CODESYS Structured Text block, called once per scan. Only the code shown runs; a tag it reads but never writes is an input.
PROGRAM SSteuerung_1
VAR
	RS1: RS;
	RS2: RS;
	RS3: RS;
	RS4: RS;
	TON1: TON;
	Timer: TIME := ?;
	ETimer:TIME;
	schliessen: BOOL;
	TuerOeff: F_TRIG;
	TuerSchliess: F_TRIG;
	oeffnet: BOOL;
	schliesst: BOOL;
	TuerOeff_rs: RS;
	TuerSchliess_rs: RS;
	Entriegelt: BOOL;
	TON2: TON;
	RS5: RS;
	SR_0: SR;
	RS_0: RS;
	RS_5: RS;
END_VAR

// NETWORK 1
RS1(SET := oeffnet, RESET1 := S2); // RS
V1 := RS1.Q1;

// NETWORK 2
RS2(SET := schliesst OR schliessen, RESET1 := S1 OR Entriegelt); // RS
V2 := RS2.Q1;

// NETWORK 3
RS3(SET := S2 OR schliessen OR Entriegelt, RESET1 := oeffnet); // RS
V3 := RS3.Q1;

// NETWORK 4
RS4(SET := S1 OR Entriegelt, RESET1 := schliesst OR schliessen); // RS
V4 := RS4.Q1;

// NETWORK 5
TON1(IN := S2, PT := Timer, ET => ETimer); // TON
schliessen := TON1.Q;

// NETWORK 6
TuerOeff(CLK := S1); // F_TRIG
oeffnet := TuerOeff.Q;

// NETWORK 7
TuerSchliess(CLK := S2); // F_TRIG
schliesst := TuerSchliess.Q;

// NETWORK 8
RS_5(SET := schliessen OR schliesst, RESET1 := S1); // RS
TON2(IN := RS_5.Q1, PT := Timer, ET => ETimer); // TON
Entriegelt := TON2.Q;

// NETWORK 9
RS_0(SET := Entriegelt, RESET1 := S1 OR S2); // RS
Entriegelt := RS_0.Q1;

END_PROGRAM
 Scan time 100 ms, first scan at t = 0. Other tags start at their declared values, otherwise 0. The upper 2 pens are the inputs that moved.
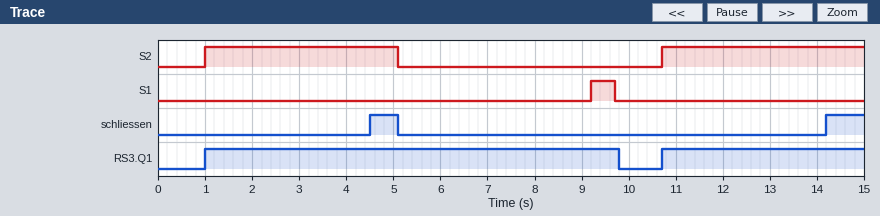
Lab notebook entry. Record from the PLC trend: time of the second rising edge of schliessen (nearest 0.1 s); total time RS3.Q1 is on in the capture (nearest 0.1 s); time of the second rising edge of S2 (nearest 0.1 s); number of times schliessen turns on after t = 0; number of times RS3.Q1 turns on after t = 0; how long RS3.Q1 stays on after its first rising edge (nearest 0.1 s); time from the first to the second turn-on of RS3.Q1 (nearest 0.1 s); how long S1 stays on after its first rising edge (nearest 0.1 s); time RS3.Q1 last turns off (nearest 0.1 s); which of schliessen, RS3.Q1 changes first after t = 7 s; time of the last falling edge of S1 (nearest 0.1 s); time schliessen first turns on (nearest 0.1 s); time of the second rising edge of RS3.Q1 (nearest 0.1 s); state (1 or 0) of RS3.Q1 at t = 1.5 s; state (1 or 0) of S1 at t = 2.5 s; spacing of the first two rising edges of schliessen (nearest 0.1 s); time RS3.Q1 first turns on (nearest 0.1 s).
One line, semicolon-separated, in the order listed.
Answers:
14.2 s; 13.1 s; 10.7 s; 2; 2; 8.8 s; 9.7 s; 0.5 s; 9.8 s; RS3.Q1; 9.7 s; 4.5 s; 10.7 s; 1; 0; 9.7 s; 1.0 s
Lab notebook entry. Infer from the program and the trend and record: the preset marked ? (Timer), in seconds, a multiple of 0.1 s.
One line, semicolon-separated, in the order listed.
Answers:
3.5 s
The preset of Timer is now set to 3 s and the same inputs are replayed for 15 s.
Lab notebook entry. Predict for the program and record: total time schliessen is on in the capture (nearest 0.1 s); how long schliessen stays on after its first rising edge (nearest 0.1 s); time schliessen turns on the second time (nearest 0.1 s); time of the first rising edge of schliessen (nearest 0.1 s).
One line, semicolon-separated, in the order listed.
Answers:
2.4 s; 1.1 s; 13.7 s; 4.0 s
